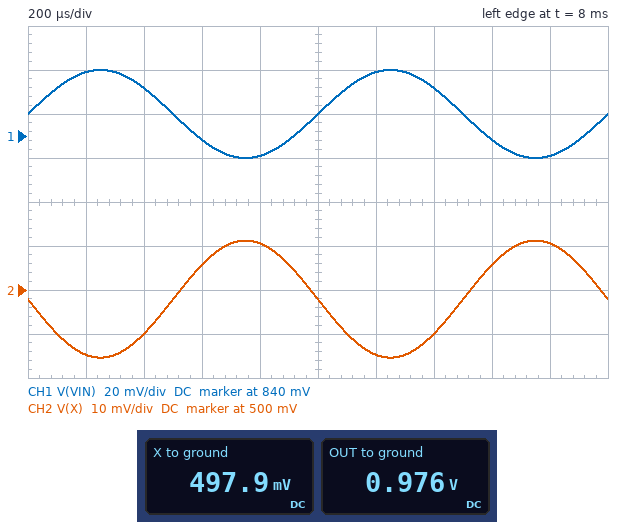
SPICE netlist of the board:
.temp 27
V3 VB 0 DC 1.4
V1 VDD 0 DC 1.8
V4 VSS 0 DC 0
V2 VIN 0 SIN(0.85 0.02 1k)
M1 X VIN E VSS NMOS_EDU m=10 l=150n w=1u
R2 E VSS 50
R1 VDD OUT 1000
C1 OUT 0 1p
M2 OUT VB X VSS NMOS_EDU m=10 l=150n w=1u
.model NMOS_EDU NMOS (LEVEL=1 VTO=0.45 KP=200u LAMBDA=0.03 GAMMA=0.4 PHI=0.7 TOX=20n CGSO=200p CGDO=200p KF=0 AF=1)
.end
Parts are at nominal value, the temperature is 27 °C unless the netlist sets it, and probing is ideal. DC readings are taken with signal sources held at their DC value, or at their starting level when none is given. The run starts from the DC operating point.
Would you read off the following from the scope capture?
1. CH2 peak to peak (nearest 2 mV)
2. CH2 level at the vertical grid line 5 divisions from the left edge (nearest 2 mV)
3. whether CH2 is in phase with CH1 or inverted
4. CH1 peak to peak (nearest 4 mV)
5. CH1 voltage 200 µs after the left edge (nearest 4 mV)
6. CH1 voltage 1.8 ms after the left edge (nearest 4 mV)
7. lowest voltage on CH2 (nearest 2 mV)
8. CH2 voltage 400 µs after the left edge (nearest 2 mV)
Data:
26 mV
498 mV
inverted
40 mV
868 mV
832 mV
484 mV
490 mV
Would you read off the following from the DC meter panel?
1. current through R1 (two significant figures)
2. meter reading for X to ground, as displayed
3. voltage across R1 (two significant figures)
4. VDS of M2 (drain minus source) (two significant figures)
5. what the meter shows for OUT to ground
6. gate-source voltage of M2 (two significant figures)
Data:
820 µA
497.9 mV
820 mV
480 mV
0.976 V
900 mV
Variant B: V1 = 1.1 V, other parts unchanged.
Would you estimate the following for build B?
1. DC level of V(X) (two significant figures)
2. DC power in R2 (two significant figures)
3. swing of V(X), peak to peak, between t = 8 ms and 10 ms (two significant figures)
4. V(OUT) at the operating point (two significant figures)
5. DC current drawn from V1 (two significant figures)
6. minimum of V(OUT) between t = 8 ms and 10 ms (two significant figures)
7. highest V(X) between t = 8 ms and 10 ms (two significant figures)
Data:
270 mV
27 µW
41 mV
360 mV
740 µA
340 mV
290 mV
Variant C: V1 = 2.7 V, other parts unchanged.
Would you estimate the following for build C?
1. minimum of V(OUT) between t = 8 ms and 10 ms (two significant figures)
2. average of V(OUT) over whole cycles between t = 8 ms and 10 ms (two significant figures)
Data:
1.8 V
1.9 V
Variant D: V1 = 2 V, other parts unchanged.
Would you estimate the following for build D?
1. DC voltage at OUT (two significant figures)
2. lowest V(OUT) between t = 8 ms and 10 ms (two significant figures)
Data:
1.2 V
1.1 V
